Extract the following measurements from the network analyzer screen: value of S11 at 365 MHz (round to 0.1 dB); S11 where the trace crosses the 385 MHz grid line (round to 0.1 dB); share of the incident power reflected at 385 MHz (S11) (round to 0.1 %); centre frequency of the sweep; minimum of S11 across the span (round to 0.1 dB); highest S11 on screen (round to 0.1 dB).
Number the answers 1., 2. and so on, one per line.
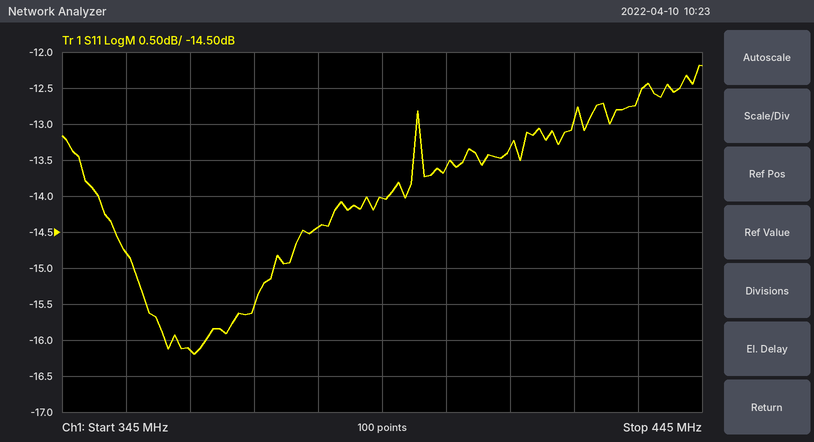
1. -16.1 dB
2. -14.4 dB
3. 3.6 %
4. 395 MHz
5. -16.2 dB
6. -12.2 dB
